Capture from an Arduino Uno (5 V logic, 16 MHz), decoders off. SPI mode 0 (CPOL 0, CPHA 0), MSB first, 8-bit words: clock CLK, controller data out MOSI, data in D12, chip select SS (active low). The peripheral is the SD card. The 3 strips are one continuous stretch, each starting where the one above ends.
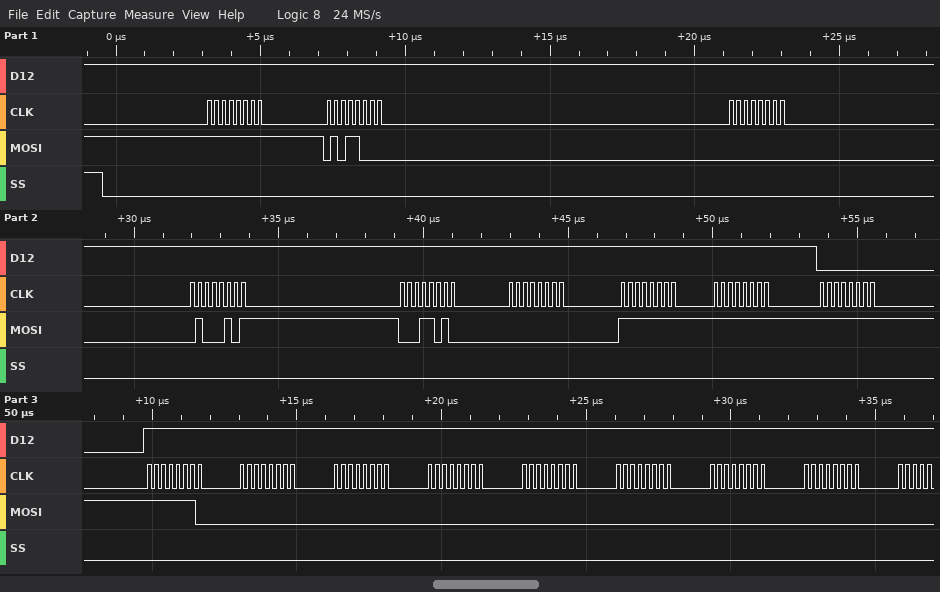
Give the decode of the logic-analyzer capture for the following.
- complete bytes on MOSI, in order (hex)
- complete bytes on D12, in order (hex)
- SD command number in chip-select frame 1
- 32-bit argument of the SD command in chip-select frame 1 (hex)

0xFF 0x58 0x00 0x45 0x1A 0x00 0xFF 0xFF 0xFF 0xFE 0x00 0x00 0x00 0x00 0x00 0x00 0x00
0xFF 0xFF 0xFF 0xFF 0xFF 0xFF 0xFF 0xFF 0x00 0xFF 0xFF 0xFF 0xFF 0xFF 0xFF 0xFF 0xFF
CMD24
0x00451A00
